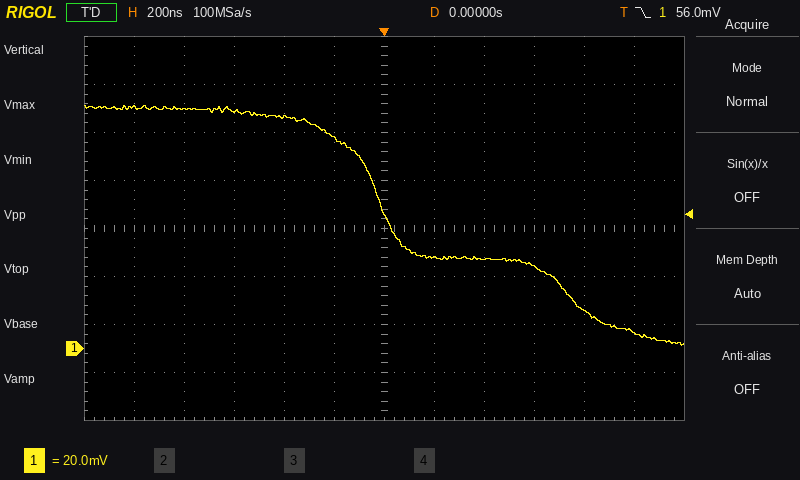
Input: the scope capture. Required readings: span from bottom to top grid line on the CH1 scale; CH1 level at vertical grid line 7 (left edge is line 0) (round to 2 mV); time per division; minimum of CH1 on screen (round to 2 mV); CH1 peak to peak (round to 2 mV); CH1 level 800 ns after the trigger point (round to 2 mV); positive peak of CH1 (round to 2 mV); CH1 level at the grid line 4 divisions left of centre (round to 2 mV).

160 mV
38 mV
200 ns
2 mV
100 mV
16 mV
102 mV
100 mV
